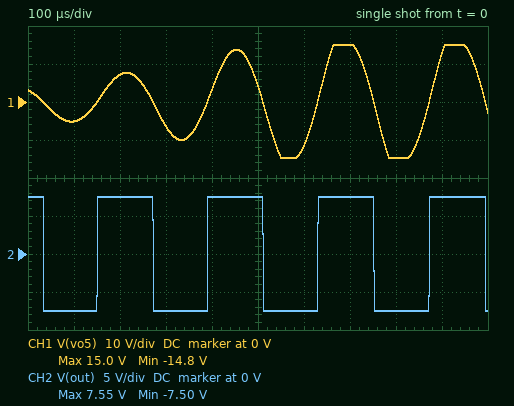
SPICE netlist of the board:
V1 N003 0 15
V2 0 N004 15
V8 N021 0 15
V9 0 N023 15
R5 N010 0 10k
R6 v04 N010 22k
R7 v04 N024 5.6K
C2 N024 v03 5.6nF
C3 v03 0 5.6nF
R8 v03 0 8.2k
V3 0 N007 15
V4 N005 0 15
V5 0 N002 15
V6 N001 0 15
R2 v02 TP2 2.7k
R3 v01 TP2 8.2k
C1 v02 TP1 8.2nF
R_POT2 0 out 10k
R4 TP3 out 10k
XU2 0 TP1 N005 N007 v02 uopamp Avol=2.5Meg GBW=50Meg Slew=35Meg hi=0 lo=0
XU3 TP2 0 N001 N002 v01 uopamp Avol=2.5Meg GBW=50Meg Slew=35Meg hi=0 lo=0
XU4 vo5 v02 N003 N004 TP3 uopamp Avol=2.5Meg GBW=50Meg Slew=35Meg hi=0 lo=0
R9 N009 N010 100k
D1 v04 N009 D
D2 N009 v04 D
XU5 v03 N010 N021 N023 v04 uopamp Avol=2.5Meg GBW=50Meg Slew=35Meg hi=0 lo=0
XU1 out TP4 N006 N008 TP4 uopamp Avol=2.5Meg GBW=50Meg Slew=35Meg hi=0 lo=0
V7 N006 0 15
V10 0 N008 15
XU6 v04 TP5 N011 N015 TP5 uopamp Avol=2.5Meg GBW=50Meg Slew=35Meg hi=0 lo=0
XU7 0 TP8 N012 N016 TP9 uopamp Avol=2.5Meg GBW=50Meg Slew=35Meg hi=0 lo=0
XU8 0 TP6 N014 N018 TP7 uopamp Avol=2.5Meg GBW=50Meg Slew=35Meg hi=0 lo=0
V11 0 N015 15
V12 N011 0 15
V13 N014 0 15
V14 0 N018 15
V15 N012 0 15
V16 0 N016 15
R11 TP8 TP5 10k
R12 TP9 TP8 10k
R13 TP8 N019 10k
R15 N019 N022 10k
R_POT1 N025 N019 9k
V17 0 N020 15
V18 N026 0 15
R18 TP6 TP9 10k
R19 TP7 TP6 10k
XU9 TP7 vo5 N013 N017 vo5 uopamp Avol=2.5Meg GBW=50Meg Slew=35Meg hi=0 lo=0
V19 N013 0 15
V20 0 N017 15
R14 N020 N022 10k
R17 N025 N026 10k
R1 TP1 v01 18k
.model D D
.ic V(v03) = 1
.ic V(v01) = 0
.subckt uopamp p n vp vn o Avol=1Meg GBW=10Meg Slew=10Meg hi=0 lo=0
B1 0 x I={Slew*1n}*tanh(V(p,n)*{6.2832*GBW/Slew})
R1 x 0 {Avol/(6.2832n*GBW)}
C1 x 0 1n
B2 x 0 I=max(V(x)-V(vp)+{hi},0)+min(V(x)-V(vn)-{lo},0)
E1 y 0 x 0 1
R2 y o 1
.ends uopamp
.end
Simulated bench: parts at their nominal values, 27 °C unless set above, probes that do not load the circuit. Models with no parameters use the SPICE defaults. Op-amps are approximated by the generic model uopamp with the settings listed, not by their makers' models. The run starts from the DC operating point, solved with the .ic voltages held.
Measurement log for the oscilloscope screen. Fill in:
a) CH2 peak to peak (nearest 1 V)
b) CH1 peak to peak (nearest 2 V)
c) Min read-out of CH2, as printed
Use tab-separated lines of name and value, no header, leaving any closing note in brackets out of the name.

CH2 peak to peak	15 V
CH1 peak to peak	30 V
Min read-out of CH2, as printed	-7.50 V
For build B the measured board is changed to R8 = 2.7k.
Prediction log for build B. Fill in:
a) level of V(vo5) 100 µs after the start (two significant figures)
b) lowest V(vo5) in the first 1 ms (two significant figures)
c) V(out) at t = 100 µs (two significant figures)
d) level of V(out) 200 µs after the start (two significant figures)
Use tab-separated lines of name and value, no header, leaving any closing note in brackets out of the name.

level of V(vo5) 100 µs after the start	480 mV
lowest V(vo5) in the first 1 ms	-1.6 V
V(out) at t = 100 µs	7.5 V
level of V(out) 200 µs after the start	-7.5 V
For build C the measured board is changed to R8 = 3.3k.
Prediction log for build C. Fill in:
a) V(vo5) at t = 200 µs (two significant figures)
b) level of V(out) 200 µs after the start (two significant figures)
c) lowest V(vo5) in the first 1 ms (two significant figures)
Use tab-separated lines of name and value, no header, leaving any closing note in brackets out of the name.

V(vo5) at t = 200 µs	-270 mV
level of V(out) 200 µs after the start	-7.5 V
lowest V(vo5) in the first 1 ms	-2.0 V
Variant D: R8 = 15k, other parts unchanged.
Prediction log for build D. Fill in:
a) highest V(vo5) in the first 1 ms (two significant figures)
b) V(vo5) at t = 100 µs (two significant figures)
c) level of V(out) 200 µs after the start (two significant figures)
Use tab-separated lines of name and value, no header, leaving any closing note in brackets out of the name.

highest V(vo5) in the first 1 ms	15 V
V(vo5) at t = 100 µs	-8.1 V
level of V(out) 200 µs after the start	-7.5 V
